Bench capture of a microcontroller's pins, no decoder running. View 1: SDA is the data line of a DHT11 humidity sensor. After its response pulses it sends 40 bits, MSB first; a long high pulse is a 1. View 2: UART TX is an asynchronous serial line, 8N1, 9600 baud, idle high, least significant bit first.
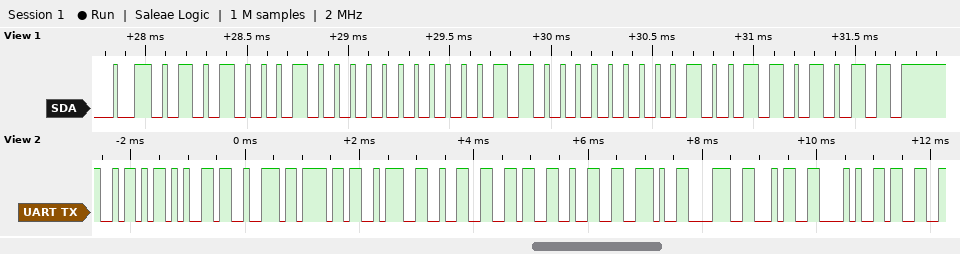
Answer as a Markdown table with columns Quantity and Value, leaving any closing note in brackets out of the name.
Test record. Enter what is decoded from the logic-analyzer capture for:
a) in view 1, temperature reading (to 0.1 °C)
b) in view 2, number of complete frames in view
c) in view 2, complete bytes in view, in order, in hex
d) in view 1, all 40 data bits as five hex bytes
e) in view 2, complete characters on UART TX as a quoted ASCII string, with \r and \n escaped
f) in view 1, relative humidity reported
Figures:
| Quantity | Value |
|---|---|
| in view 1, temperature reading | 24.2 °C |
| in view 2, number of complete frames in view | 13 |
| in view 2, complete bytes in view, in order, in hex | 0x5A 0x65 0x72 0x6F 0x3A 0x32 0x36 0x32 0x2E 0x38 0x34 0x28 0x33 |
| in view 1, all 40 data bits as five hex bytes | 51 00 18 02 6B |
| in view 2, complete characters on UART TX as a quoted ASCII string, with \r and \n escaped | "Zero:262.84(3" |
| in view 1, relative humidity reported | 81 % |
